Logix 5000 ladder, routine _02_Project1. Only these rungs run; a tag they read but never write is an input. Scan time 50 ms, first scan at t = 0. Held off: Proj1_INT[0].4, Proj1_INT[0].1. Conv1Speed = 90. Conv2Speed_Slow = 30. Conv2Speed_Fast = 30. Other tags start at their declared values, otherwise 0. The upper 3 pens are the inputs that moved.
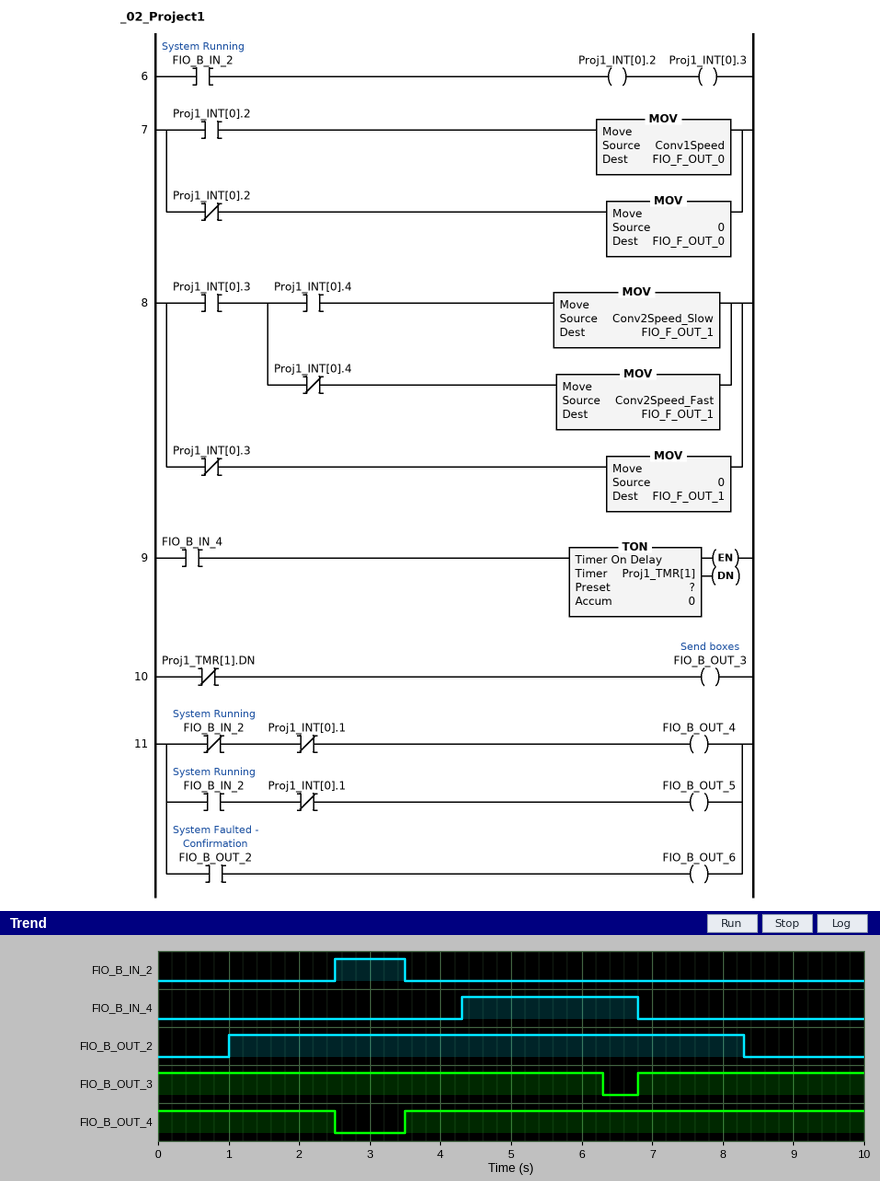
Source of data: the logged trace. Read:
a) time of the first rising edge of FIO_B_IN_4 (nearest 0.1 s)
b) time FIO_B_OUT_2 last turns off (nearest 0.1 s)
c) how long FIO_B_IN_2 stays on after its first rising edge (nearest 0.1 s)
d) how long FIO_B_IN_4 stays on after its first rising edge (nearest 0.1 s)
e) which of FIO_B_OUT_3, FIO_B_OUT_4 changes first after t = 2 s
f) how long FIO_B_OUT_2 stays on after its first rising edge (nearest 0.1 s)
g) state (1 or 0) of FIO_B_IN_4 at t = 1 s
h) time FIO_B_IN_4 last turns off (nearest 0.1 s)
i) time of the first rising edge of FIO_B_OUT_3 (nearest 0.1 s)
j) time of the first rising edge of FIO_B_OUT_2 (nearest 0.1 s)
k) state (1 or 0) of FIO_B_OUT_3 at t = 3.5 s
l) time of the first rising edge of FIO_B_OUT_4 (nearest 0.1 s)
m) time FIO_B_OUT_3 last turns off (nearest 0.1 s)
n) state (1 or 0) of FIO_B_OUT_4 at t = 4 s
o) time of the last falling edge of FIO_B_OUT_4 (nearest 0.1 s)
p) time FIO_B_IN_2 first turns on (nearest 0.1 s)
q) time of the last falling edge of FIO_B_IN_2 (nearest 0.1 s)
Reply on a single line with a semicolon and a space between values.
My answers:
4.3 s; 8.3 s; 1.0 s; 2.5 s; FIO_B_OUT_4; 7.3 s; 0; 6.8 s; 6.8 s; 1.0 s; 1; 3.5 s; 6.3 s; 1; 2.5 s; 2.5 s; 3.5 s
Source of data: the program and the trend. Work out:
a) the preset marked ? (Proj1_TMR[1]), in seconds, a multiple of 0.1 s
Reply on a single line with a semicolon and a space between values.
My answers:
2.0 s
